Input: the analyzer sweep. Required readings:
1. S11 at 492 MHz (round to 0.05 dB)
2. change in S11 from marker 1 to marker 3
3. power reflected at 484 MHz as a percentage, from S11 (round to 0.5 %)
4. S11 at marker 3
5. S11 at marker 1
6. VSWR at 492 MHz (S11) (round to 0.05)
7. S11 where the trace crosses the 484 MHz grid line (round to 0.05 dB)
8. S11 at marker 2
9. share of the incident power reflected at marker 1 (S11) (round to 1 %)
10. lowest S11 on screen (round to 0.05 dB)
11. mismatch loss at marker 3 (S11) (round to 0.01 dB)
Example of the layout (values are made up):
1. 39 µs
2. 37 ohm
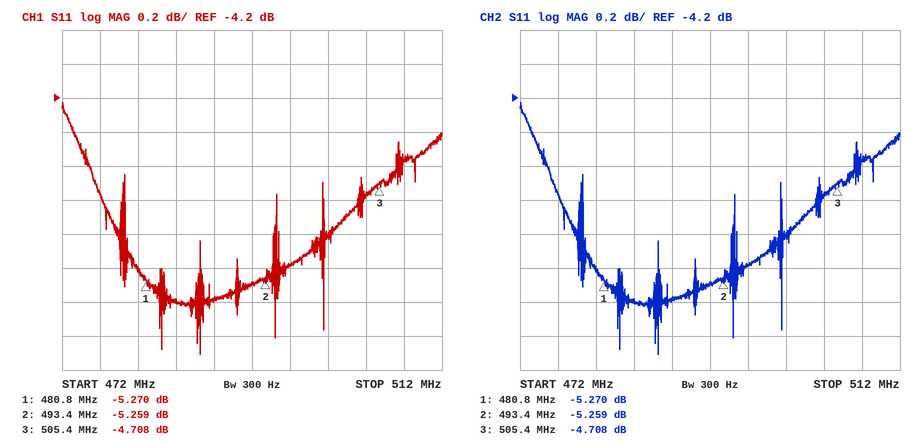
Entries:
1. -5.30 dB
2. 0.562 dB
3. 29.0 %
4. -4.708 dB
5. -5.270 dB
6. 3.40
7. -5.40 dB
8. -5.259 dB
9. 30 %
10. -5.70 dB
11. 1.79 dB
